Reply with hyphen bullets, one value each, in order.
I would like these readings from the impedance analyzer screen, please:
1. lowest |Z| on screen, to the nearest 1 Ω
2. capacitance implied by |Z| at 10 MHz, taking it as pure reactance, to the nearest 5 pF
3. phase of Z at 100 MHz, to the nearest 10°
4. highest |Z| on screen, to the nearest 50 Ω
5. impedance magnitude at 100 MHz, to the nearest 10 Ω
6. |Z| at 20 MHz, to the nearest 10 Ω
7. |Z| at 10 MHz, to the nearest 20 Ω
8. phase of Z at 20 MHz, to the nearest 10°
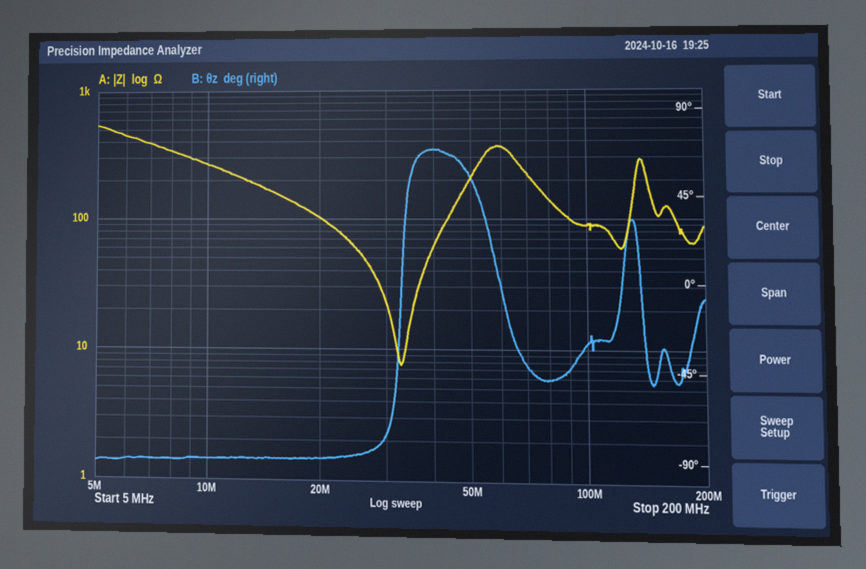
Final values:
- 8 Ω
- 60 pF
- -30°
- 550 Ω
- 90 Ω
- 100 Ω
- 260 Ω
- -90°
